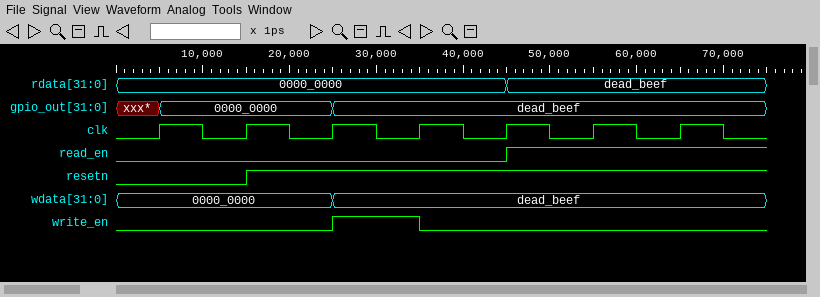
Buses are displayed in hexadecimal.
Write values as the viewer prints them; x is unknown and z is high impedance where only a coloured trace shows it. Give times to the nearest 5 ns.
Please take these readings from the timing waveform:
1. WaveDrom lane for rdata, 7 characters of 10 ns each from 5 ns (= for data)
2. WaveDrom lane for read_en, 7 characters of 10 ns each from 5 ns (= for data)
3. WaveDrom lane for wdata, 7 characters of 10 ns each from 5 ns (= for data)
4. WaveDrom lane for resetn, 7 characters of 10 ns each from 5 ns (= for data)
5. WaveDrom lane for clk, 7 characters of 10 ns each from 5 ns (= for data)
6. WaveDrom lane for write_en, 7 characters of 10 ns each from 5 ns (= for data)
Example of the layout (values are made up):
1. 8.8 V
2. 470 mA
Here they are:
1. {name: 'rdata', wave: '=...=..', data: '0000_0000 dead_beef'}
2. {name: 'read_en', wave: '0...1..'}
3. {name: 'wdata', wave: '=.=....', data: '0000_0000 dead_beef'}
4. {name: 'resetn', wave: '01.....'}
5. {name: 'clk', wave: 'p......'}
6. {name: 'write_en', wave: '0.10...'}
